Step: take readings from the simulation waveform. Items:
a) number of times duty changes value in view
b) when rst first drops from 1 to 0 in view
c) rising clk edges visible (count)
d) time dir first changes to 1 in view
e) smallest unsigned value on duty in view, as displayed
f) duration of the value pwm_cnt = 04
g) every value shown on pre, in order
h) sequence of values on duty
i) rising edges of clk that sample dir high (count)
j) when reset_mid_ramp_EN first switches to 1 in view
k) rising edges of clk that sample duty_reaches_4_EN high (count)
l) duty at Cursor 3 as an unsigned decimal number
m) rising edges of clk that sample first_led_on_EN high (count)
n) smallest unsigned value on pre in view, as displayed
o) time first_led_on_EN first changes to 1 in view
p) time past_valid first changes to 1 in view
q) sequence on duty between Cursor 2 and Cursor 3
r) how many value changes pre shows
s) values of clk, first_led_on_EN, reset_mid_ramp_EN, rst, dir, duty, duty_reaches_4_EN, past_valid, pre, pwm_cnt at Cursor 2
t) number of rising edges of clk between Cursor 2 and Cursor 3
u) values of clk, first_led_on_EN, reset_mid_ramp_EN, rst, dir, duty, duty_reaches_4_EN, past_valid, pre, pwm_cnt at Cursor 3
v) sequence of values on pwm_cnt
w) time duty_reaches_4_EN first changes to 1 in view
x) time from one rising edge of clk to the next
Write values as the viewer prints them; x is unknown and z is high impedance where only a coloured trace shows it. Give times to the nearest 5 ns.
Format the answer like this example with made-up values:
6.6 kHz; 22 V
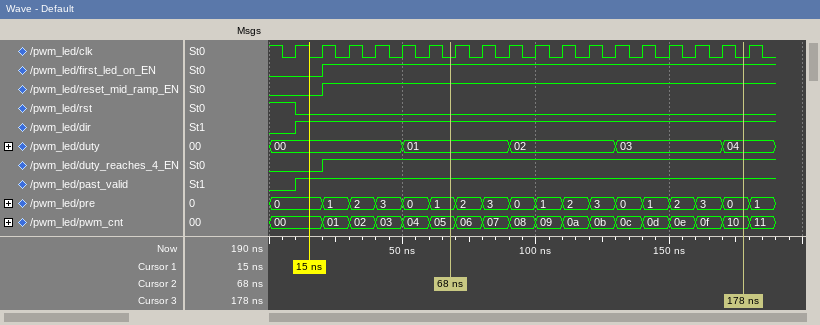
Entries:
4; 10 ns; 18; 10 ns; 00; 10 ns; 0, 1, 2, 3, 0, 1, 2, 3, 0, 1, 2, 3, 0, 1, 2, 3, 0, 1; 00, 01, 02, 03, 04; 17; 20 ns; 16; 4; 16; 0; 20 ns; 10 ns; 01, 02, 03, 04; 17; clk=0, first_led_on_EN=1, reset_mid_ramp_EN=1, rst=0, dir=1, duty=01, duty_reaches_4_EN=1, past_valid=1, pre=1, pwm_cnt=05; 11; clk=0, first_led_on_EN=1, reset_mid_ramp_EN=1, rst=0, dir=1, duty=04, duty_reaches_4_EN=1, past_valid=1, pre=0, pwm_cnt=10; 00, 01, 02, 03, 04, 05, 06, 07, 08, 09, 0a, 0b, 0c, 0d, 0e, 0f, 10, 11; 20 ns; 10 ns
